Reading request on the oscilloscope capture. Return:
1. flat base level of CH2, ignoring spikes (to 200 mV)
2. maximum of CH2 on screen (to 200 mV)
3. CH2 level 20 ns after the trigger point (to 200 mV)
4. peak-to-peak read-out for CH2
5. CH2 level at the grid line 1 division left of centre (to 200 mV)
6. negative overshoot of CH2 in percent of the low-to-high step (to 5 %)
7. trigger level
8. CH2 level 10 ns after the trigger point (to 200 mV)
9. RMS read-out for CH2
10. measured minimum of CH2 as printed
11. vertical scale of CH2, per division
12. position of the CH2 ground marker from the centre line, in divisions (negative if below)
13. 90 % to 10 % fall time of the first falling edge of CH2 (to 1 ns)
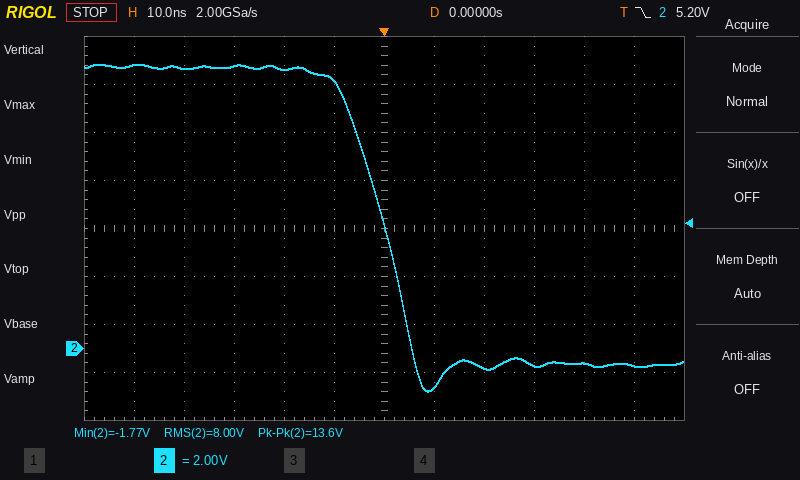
-600 mV
11.8 V
-800 mV
13.6 V
11.2 V
10 %
5.20 V
-1.6 V
8.00 V
-1.77 V
2 V
-2.5 div
13 ns
